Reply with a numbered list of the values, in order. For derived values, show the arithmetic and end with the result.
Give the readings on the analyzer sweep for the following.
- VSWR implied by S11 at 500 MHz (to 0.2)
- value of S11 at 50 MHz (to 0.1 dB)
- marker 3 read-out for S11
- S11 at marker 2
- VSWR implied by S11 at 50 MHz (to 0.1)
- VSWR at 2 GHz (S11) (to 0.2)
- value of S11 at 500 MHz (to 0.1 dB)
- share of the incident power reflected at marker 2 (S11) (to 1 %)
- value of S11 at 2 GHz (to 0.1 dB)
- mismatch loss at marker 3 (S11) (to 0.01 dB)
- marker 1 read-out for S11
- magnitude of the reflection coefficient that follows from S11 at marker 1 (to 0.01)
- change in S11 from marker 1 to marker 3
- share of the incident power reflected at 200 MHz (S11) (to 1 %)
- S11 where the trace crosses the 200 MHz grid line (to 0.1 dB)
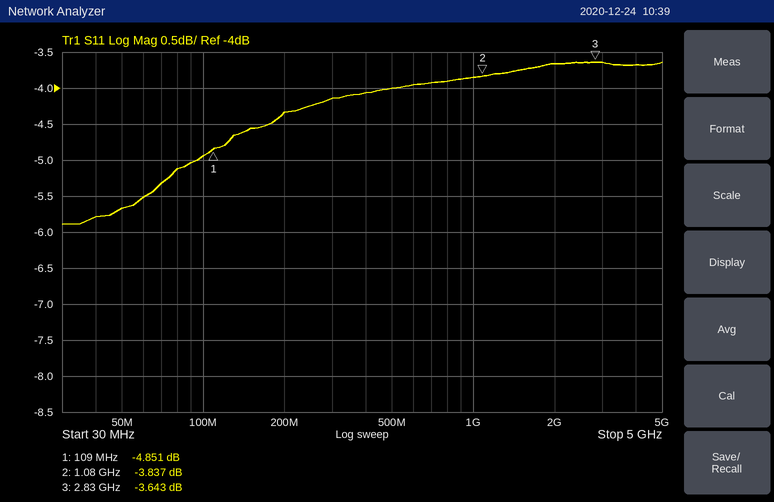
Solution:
1. |Γ| = 10^(-4/20) = 0.6310; VSWR = (1 + 0.6310)/(1 − 0.6310) ≈ 4.4
2. -5.7 dB
3. -3.643 dB
4. -3.837 dB
5. |Γ| = 10^(-5.7/20) = 0.5188; VSWR = (1 + 0.5188)/(1 − 0.5188) ≈ 3.2
6. |Γ| = 10^(-3.7/20) = 0.6531; VSWR = (1 + 0.6531)/(1 − 0.6531) ≈ 4.8
7. -4.0 dB
8. 10^(-3.837/10) ≈ 41 %
9. -3.7 dB
10. −10 log10(1 − 10^(-3.643/10)) ≈ 2.46 dB
11. -4.851 dB
12. 10^(-4.851/20) ≈ 0.57
13. -3.643 − (-4.851) = 1.208 dB
14. 10^(-4.3/10) ≈ 37 %
15. -4.3 dB
